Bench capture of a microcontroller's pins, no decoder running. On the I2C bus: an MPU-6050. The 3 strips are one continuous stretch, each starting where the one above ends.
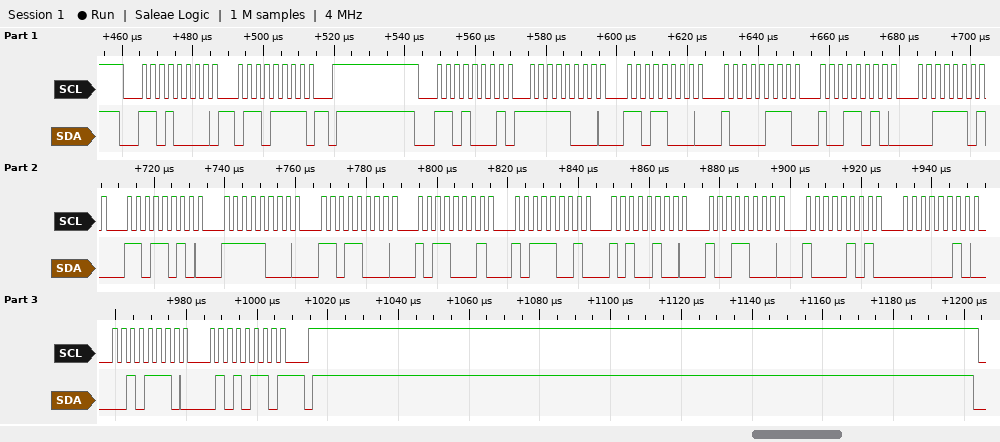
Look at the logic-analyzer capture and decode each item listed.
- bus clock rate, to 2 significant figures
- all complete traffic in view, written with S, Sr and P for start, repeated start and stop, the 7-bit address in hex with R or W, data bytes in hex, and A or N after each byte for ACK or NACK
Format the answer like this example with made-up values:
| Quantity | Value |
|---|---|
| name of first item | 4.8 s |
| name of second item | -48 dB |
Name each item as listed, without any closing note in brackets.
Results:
| Quantity | Value |
|---|---|
| bus clock rate, to 2 significant figures | 400 kHz |
| all complete traffic in view, written with S, Sr and P for start, repeated start and stop, the 7-bit address in hex with R or W, data bytes in hex, and A or N after each byte for ACK or NACK | S 68W A 6F A P S 68R A F8 A D8 A 87 A 9A A 3D A DA A F8 A D8 A B1 A B9 A A4 A 98 A 85 A 02 A 2E A 56 N P |
